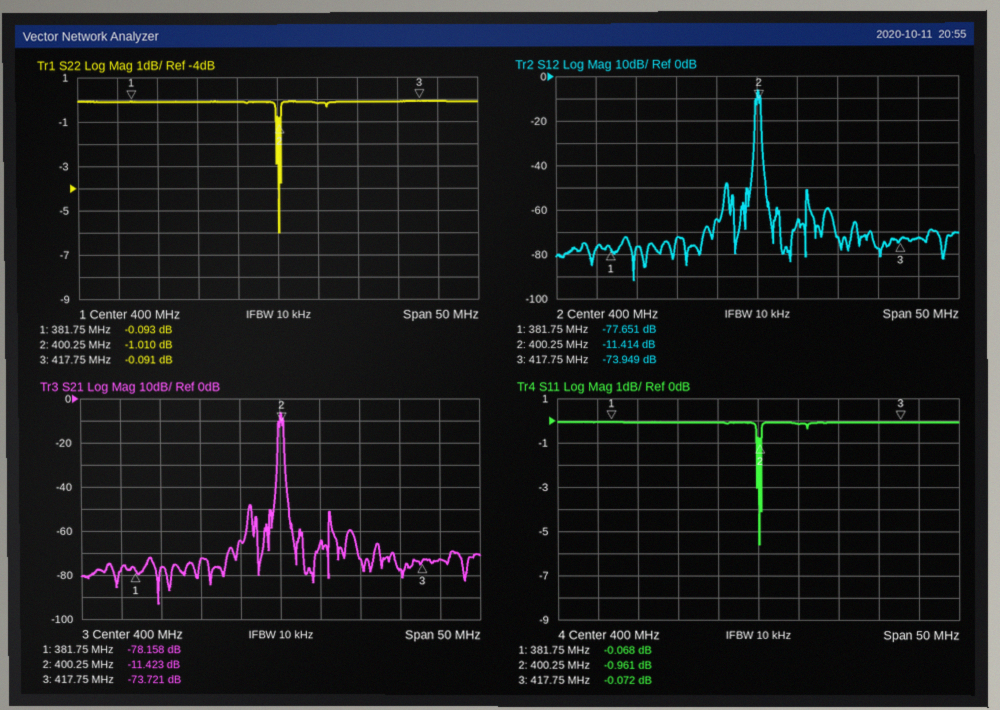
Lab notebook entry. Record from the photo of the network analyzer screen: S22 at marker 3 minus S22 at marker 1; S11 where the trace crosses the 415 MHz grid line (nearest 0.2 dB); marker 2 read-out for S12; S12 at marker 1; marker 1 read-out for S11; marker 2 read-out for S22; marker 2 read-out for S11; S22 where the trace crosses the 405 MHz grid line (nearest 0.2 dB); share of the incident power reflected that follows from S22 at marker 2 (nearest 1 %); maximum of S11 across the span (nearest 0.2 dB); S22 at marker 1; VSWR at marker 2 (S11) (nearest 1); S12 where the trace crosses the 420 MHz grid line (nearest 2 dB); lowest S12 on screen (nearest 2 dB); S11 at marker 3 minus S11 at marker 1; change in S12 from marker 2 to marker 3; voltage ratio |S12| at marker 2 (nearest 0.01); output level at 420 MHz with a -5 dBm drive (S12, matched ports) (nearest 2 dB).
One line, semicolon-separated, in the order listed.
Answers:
0.002 dB; 0.0 dB; -11.414 dB; -77.651 dB; -0.068 dB; -1.010 dB; -0.961 dB; -0.2 dB; 79 %; 0.0 dB; -0.093 dB; 18; -72 dB; -92 dB; -0.004 dB; -62.535 dB; 0.27; -78 dBm
